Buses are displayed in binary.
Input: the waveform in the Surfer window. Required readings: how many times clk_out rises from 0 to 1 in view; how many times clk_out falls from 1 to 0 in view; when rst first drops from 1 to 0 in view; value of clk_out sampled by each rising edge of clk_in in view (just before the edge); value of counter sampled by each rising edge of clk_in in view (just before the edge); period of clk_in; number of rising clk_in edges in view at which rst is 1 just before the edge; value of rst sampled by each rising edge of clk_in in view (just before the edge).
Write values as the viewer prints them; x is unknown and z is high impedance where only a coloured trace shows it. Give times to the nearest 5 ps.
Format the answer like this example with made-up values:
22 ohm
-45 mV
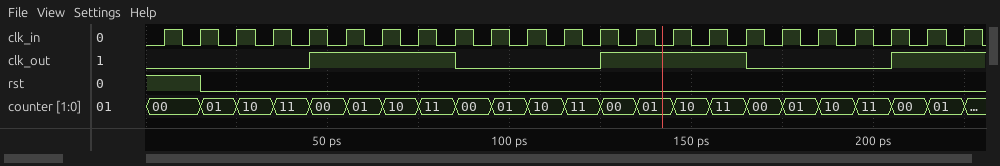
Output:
3
2
15 ps
0 0 0 0 0 1 1 1 1 0 0 0 0 1 1 1 1 0 0 0 0 1 1
00, 00, 01, 10, 11, 00, 01, 10, 11, 00, 01, 10, 11, 00, 01, 10, 11, 00, 01, 10, 11, 00, 01
10 ps
2
1 1 0 0 0 0 0 0 0 0 0 0 0 0 0 0 0 0 0 0 0 0 0
